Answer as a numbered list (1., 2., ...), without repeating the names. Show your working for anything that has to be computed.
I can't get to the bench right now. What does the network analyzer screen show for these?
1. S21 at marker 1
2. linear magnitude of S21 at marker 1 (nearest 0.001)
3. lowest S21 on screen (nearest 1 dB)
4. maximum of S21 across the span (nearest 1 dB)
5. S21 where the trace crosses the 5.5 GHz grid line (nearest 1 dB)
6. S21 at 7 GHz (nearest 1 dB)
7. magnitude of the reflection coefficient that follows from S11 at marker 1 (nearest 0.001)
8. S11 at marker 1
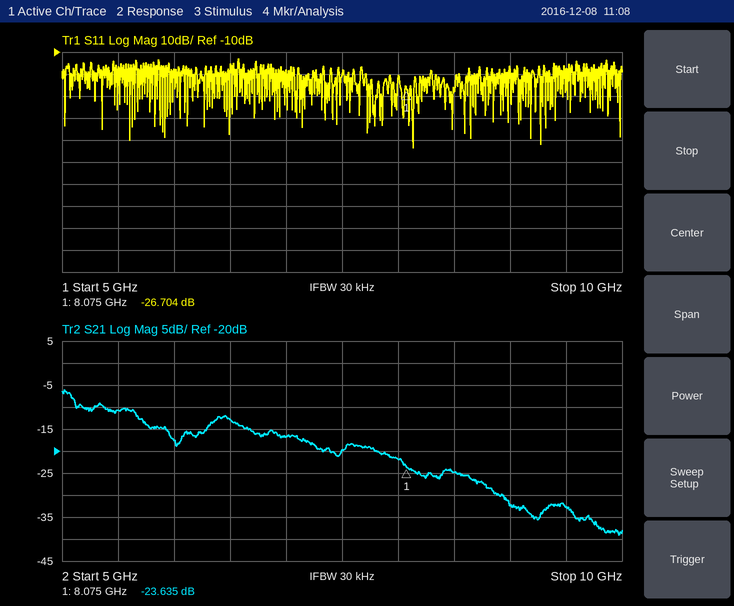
1. -23.635 dB
2. 10^(-23.635/20) ≈ 0.066
3. -39 dB
4. -6 dB
5. -11 dB
6. -17 dB
7. 10^(-26.704/20) ≈ 0.046
8. -26.704 dB
